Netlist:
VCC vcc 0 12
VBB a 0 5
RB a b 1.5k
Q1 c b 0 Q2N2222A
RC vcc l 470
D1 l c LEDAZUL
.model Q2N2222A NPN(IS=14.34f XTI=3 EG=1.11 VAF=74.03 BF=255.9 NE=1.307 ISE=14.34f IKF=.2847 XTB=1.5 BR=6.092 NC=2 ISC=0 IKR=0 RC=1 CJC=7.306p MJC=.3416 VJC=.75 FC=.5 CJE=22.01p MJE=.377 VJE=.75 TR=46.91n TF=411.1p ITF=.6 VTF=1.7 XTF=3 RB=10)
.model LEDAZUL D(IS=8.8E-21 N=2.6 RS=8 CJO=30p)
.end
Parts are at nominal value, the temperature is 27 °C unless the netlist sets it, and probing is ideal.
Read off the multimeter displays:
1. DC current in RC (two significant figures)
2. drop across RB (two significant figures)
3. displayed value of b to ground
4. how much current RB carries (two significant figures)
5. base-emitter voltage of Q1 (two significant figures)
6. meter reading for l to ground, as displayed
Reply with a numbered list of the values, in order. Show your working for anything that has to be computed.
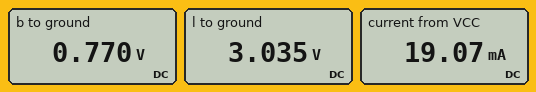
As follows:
1. (12 V - 3.035 V) / 470 Ω = 19 mA
2. 5 V - 770 mV = 4.2 V
3. 0.770 V
4. (5 V - 770 mV) / 1.5 kΩ = 2.8 mA
5. 770 mV = 770 mV
6. 3.035 V
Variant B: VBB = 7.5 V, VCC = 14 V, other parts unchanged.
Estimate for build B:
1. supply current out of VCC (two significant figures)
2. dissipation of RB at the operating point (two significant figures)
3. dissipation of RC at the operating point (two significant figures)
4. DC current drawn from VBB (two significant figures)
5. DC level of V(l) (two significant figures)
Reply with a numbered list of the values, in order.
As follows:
1. 23 mA
2. 30 mW
3. 250 mW
4. 4.5 mA
5. 3.1 V
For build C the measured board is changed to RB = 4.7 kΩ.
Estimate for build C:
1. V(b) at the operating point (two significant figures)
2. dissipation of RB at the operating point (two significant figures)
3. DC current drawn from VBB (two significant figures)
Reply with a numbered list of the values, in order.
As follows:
1. 740 mV
2. 3.9 mW
3. 910 µA
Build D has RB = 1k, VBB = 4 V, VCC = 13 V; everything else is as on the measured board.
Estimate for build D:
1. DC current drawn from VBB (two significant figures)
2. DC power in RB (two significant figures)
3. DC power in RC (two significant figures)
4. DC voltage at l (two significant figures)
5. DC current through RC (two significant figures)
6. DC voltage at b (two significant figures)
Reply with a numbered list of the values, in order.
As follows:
1. 3.2 mA
2. 10 mW
3. 210 mW
4. 3.1 V
5. 21 mA
6. 780 mV
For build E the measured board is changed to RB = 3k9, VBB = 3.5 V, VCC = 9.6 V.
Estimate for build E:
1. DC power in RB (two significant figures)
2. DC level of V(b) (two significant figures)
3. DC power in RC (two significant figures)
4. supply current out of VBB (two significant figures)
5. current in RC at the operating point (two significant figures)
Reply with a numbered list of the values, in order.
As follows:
1. 2.0 mW
2. 730 mV
3. 93 mW
4. 710 µA
5. 14 mA
